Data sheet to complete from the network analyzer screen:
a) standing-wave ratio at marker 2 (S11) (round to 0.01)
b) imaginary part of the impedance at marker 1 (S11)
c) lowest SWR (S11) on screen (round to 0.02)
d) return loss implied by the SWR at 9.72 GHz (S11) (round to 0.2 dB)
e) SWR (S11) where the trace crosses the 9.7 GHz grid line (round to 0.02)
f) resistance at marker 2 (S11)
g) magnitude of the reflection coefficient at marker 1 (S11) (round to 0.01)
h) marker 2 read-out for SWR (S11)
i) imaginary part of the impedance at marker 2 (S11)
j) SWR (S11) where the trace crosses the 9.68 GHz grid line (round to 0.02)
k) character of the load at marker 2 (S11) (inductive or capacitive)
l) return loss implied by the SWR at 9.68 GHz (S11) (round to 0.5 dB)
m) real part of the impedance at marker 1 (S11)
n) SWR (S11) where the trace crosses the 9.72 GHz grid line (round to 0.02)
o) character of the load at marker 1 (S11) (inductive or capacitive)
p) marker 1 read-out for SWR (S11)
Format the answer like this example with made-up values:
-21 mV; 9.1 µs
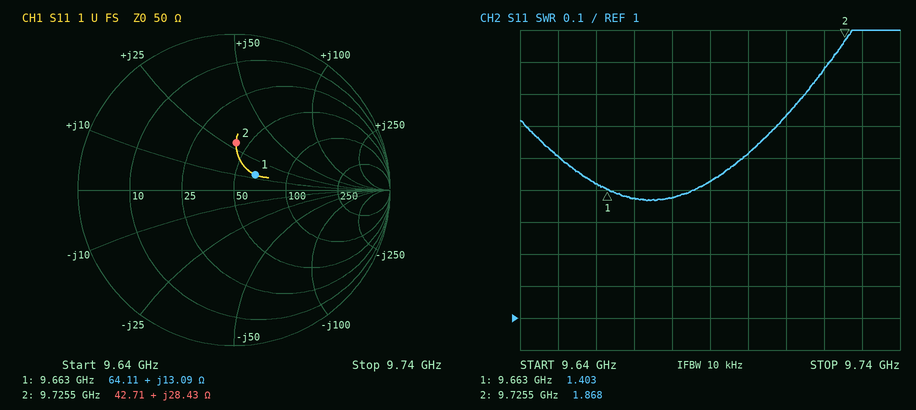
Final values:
1.87; +13.09 Ω; 1.36; 11.0 dB; 1.52; 42.71 Ω; 0.17; 1.868; +28.43 Ω; 1.38; inductive; 16.0 dB; 64.11 Ω; 1.78; inductive; 1.403
